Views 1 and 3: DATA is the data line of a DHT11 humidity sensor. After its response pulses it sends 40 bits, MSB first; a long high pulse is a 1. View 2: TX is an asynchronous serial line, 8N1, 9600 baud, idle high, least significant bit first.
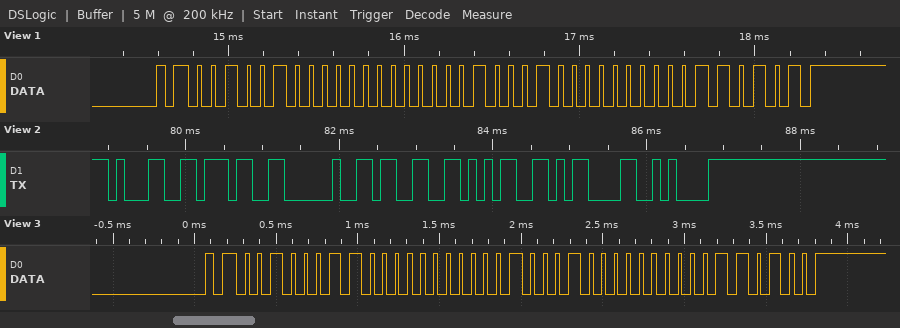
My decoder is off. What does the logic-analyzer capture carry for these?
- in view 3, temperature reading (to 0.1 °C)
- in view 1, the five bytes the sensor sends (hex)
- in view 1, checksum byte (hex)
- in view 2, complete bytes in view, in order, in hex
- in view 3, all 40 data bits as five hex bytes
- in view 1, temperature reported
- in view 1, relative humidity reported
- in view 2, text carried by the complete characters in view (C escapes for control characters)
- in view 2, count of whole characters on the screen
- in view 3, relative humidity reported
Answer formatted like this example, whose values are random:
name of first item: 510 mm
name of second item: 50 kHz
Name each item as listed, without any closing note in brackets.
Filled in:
in view 3, temperature reading: 17.0 °C
in view 1, the five bytes the sensor sends: 24 00 11 00 35
in view 1, checksum byte: 0x35
in view 2, complete bytes in view, in order, in hex: 0x31 0x37 0x20 0x33 0x35 0x0D 0x0A
in view 3, all 40 data bits as five hex bytes: 23 00 11 00 34
in view 1, temperature reported: 17.0 °C
in view 1, relative humidity reported: 36 %
in view 2, text carried by the complete characters in view: "17 35\r\n"
in view 2, count of whole characters on the screen: 7
in view 3, relative humidity reported: 35 %
